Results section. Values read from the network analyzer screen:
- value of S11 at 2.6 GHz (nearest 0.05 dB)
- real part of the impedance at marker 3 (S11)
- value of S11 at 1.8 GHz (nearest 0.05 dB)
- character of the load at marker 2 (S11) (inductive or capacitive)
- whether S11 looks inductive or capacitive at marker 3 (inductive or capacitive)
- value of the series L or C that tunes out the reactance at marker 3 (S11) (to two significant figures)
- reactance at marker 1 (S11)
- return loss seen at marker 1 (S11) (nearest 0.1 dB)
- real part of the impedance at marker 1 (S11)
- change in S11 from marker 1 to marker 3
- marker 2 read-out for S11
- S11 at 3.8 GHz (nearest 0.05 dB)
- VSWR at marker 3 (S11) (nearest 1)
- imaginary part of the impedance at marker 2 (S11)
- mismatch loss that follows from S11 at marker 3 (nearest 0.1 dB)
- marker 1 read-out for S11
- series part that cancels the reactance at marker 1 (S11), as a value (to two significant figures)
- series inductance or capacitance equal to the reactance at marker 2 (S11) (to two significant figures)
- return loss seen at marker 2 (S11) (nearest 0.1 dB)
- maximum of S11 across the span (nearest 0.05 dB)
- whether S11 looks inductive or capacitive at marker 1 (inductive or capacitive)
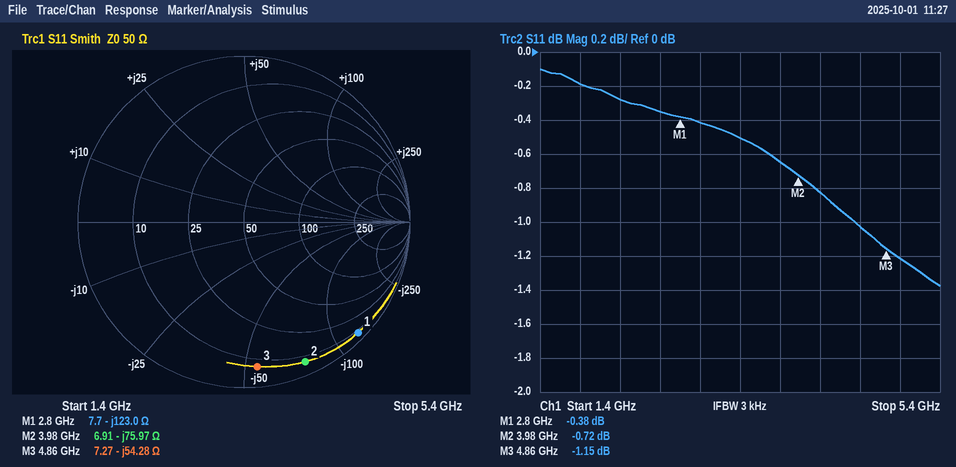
-0.35 dB
7.27 Ω
-0.20 dB
capacitive
capacitive
1.8 nH
-123.0 Ω
0.4 dB
7.7 Ω
-0.77 dB
-0.72 dB
-0.65 dB
15
-75.97 Ω
6.3 dB
-0.38 dB
7.0 nH
530 fF
0.7 dB
-0.10 dB
capacitive
